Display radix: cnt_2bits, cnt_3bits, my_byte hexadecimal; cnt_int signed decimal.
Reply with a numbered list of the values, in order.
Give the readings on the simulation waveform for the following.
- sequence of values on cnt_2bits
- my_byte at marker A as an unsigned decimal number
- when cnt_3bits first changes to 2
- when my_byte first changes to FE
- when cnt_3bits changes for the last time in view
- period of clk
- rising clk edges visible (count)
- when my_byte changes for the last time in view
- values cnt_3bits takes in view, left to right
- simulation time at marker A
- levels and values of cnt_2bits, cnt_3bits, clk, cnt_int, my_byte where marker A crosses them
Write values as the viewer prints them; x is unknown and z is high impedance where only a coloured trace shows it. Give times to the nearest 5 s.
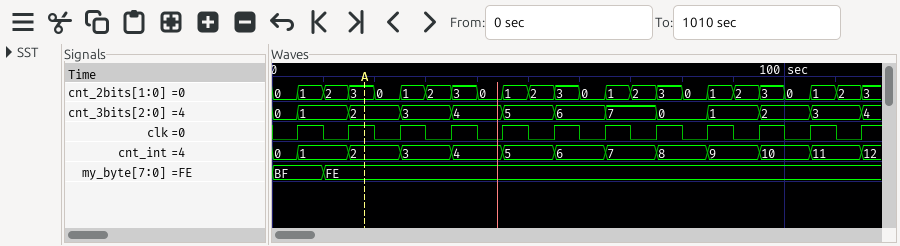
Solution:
1. 0, 1, 2, 3, 0, 1, 2, 3, 0, 1, 2, 3, 0, 1, 2, 3, 0, 1, 2, 3, 0, 1, 2, 3
2. 254
3. 15 s
4. 10 s
5. 115 s
6. 10 s
7. 12
8. 10 s
9. 0, 1, 2, 3, 4, 5, 6, 7, 0, 1, 2, 3, 4
10. 20 s
11. cnt_2bits=3, cnt_3bits=2, clk=1, cnt_int=2, my_byte=FE
